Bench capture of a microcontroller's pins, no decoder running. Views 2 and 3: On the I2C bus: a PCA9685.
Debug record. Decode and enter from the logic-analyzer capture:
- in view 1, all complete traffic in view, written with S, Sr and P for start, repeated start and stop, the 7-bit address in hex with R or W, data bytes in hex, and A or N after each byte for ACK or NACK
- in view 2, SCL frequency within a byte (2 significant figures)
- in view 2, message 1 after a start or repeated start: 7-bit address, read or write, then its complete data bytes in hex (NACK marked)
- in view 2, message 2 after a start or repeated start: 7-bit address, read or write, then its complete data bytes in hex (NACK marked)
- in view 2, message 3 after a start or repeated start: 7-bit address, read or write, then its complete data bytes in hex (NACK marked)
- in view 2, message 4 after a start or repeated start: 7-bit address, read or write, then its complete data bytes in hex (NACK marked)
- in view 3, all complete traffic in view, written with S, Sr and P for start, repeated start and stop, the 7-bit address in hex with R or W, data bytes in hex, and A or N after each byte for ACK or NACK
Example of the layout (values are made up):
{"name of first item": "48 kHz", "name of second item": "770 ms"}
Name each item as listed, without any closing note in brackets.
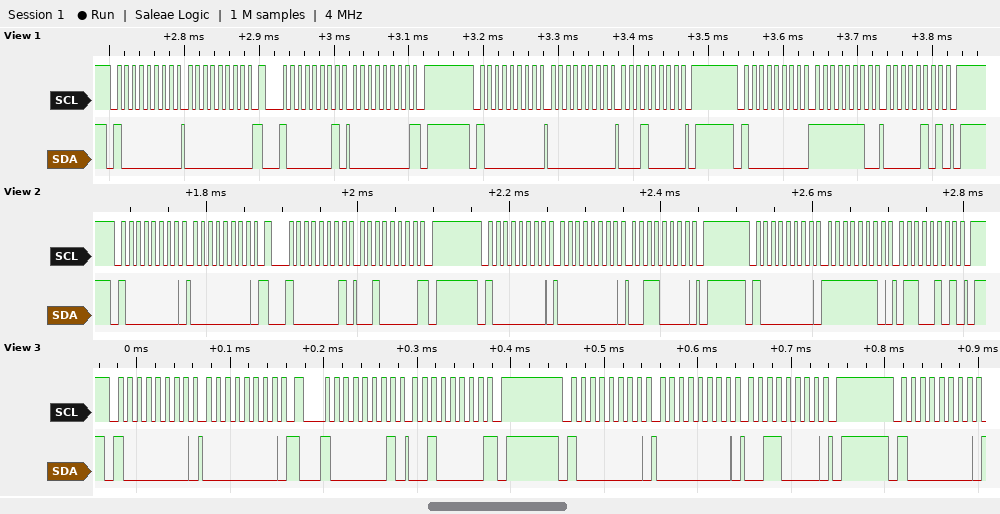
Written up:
{"in view 1, all complete traffic in view, written with S, Sr and P for start, repeated start and stop, the 7-bit address in hex with R or W, data bytes in hex, and A or N after each byte for ACK or NACK": "S 40W A 00 A Sr 40R A 00 N P S 40W A 00 A 10 A P S 40W A FE A 05 A P", "in view 2, SCL frequency within a byte": "100 kHz", "in view 2, message 1 after a start or repeated start: 7-bit address, read or write, then its complete data bytes in hex": "0x40 write: 00", "in view 2, message 2 after a start or repeated start: 7-bit address, read or write, then its complete data bytes in hex": "0x40 read: 20 NACK", "in view 2, message 3 after a start or repeated start: 7-bit address, read or write, then its complete data bytes in hex": "0x40 write: 00 30", "in view 2, message 4 after a start or repeated start: 7-bit address, read or write, then its complete data bytes in hex": "0x40 write: FE 65", "in view 3, all complete traffic in view, written with S, Sr and P for start, repeated start and stop, the 7-bit address in hex with R or W, data bytes in hex, and A or N after each byte for ACK or NACK": "S 40W A 00 A Sr 40R A 20 N P S 40W A 00 A 30 A P S 40W A"}
